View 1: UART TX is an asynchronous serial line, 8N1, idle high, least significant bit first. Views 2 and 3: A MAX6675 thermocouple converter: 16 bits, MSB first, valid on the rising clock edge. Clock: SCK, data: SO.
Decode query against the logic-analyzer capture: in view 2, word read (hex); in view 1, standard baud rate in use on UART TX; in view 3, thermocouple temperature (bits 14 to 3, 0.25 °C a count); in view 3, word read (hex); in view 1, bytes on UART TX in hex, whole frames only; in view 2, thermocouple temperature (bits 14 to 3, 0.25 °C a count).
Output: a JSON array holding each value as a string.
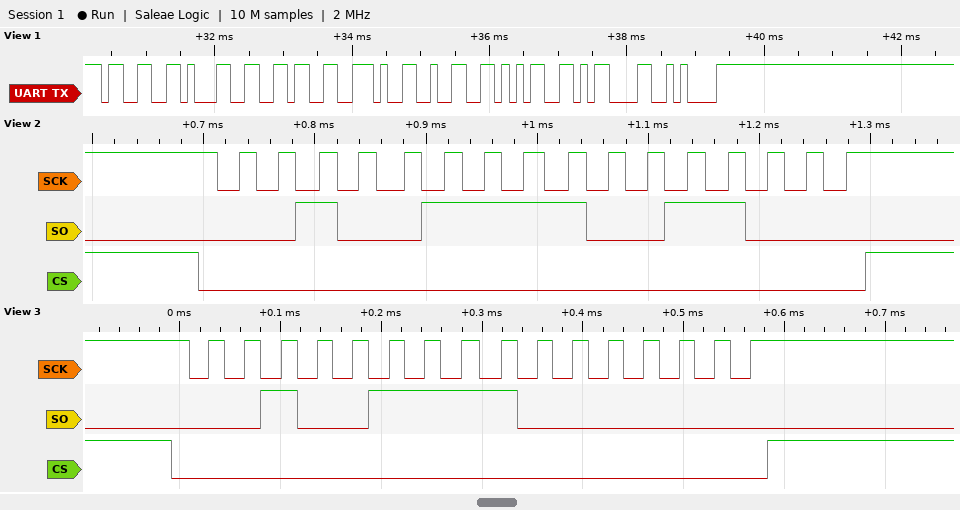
["0x2798", "9600 baud", "316.00 °C", "0x2780", "0x33 0x31 0x36 0x2E 0x32 0x35 0x0D 0x0A", "316.75 °C"]
